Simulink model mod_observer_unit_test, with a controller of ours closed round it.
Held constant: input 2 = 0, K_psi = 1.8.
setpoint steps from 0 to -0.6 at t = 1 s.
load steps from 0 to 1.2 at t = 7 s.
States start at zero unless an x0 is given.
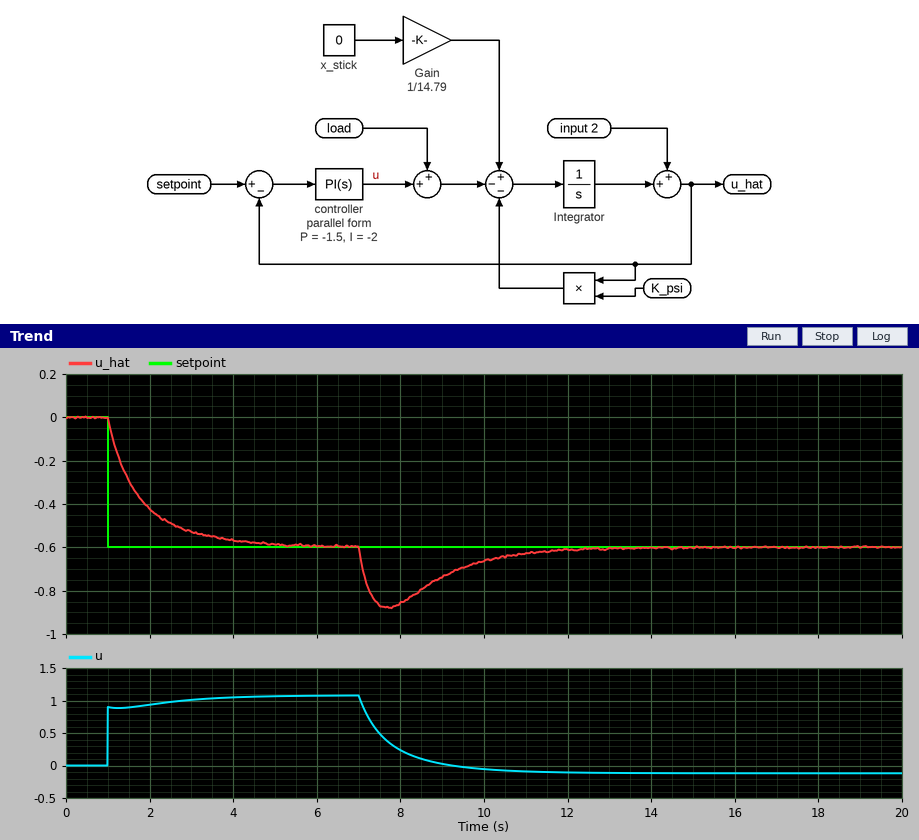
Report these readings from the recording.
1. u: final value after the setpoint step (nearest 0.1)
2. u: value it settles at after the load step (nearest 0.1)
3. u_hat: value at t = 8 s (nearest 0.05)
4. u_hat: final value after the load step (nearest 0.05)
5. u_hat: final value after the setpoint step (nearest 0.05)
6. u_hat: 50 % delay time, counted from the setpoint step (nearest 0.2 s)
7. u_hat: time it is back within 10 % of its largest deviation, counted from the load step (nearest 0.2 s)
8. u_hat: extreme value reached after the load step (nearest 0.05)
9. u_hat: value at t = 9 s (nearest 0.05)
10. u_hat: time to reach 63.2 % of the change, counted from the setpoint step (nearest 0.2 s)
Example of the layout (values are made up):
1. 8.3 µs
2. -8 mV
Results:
1. 1.1
2. -0.1
3. -0.85
4. -0.60
5. -0.60
6. 0.6 s
7. 4.0 s
8. -0.90
9. -0.75
10. 0.8 s
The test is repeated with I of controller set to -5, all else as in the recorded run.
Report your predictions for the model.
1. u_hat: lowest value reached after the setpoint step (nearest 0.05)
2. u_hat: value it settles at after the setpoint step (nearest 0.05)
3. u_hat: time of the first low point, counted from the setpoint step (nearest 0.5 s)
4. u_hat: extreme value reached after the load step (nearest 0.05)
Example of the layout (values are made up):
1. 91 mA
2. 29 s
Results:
1. -0.65
2. -0.60
3. 1.5 s
4. -0.85
